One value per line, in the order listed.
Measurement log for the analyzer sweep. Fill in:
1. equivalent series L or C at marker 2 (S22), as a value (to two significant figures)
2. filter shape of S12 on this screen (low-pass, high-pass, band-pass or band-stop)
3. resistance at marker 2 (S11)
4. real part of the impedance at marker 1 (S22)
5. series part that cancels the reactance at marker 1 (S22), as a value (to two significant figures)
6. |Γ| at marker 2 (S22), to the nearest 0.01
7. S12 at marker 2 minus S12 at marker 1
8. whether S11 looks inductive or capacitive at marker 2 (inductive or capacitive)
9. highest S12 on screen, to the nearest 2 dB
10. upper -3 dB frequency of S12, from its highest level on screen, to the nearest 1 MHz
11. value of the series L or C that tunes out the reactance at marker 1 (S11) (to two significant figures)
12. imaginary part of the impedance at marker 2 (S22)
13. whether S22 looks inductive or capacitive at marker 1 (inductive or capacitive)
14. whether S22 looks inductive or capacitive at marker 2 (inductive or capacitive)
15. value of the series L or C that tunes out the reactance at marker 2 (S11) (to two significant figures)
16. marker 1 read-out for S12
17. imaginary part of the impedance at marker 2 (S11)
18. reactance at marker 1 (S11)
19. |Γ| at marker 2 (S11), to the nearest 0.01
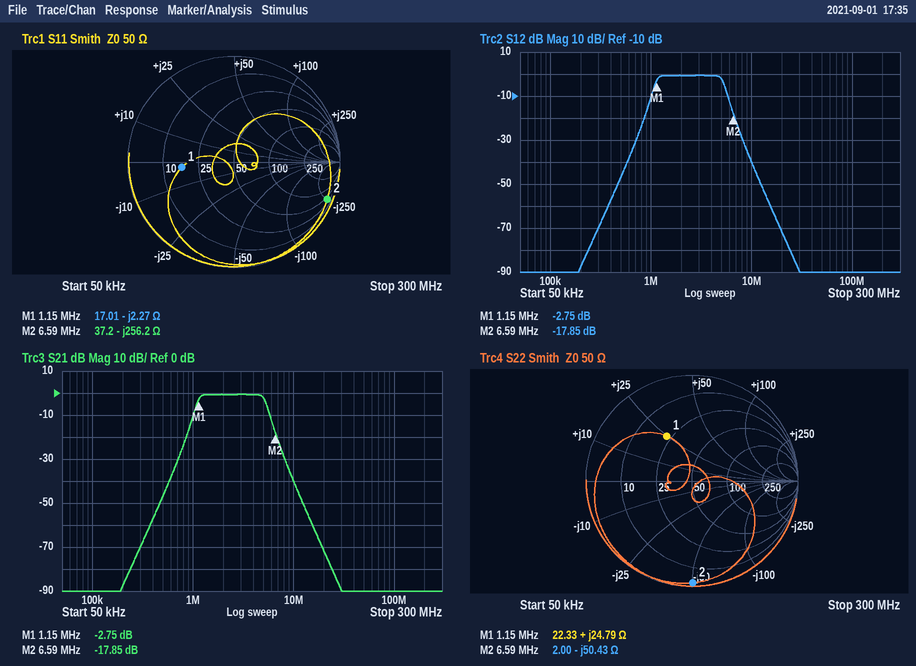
480 pF
band-pass
37.2 Ω
22.33 Ω
5.6 nF
0.96
-15.10 dB
capacitive
0 dB
5 MHz
310 nH
-50.43 Ω
inductive
capacitive
6.2 µH
-2.75 dB
-256.2 Ω
-2.27 Ω
0.95
